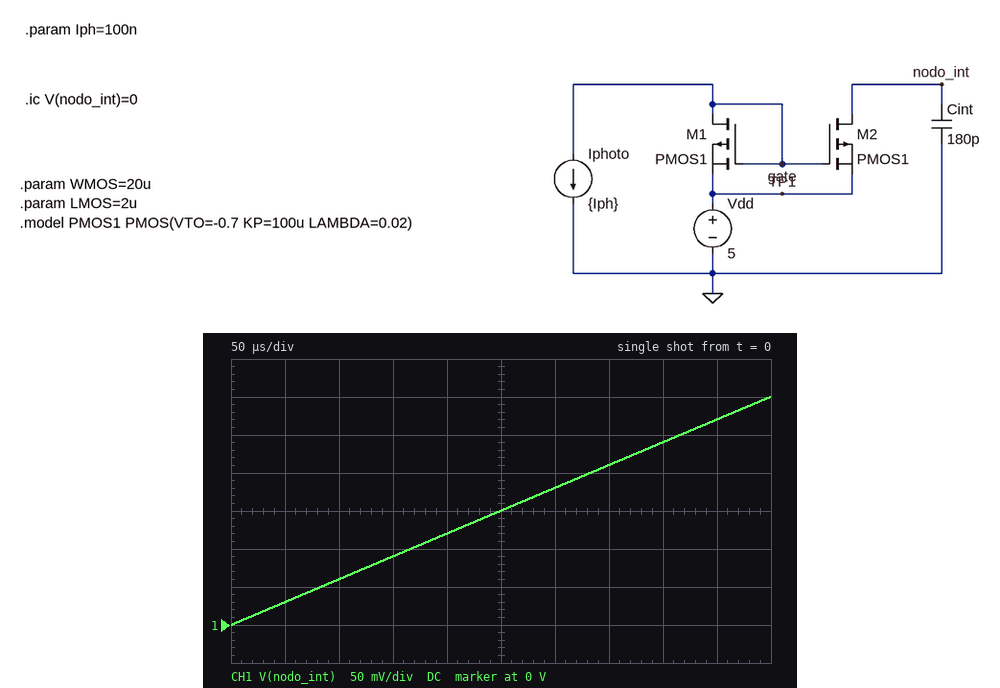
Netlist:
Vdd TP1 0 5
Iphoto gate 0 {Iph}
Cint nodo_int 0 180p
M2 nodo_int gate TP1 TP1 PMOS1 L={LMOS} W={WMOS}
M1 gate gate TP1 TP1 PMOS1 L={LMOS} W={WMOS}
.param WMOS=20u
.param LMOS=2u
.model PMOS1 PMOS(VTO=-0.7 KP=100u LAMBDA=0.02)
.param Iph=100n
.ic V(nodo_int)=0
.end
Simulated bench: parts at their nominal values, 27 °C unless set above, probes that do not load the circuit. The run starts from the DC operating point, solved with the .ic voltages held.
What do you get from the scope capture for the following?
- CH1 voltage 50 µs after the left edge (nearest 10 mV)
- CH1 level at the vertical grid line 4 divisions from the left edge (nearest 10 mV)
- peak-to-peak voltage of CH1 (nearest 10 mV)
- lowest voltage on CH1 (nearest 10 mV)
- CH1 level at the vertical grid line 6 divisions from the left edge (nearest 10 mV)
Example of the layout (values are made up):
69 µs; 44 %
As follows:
30 mV; 120 mV; 300 mV; 0 V; 180 mV
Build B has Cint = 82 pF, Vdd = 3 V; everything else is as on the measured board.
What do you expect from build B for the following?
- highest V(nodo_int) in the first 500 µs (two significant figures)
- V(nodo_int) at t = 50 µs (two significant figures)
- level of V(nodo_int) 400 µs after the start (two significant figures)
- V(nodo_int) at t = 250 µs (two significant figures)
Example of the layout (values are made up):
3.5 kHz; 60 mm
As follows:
630 mV; 64 mV; 510 mV; 320 mV
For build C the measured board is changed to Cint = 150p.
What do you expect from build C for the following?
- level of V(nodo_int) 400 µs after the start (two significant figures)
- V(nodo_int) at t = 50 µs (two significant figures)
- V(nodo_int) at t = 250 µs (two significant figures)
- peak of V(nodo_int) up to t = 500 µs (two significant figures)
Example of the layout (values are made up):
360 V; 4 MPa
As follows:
290 mV; 36 mV; 180 mV; 360 mV
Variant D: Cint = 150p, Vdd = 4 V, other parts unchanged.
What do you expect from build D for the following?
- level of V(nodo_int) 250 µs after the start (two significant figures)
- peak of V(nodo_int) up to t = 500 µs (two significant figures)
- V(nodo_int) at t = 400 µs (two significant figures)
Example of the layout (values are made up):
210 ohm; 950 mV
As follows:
180 mV; 350 mV; 280 mV
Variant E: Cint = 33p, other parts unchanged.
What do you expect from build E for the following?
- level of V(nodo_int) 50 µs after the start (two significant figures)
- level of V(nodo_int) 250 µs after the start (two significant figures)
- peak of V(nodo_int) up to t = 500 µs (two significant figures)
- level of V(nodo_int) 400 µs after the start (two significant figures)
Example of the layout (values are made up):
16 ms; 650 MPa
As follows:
160 mV; 820 mV; 1.6 V; 1.3 V
